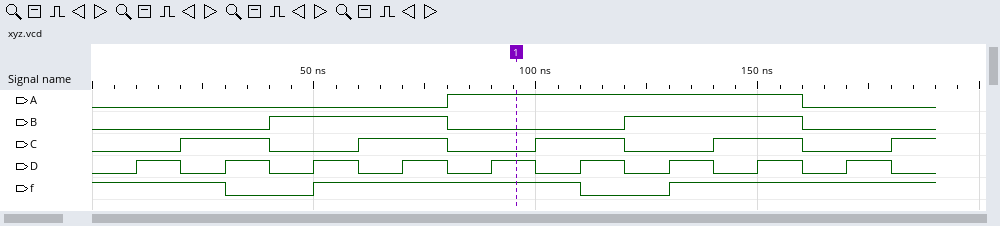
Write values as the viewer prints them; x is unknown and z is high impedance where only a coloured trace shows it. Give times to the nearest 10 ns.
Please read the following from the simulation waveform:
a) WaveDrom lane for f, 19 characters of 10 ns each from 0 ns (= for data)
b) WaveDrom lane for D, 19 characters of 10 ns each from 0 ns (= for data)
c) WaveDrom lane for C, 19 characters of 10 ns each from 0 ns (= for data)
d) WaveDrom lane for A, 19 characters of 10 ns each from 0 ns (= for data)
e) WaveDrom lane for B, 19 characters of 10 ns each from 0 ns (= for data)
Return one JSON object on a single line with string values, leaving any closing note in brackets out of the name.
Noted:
{"WaveDrom lane for f, 19 characters of 10 ns each from 0 ns": "{name: 'f', wave: '1..0.1.....0.1.....'}", "WaveDrom lane for D, 19 characters of 10 ns each from 0 ns": "{name: 'D', wave: '0101010101010101010'}", "WaveDrom lane for C, 19 characters of 10 ns each from 0 ns": "{name: 'C', wave: '0.1.0.1.0.1.0.1.0.1'}", "WaveDrom lane for A, 19 characters of 10 ns each from 0 ns": "{name: 'A', wave: '0.......1.......0..'}", "WaveDrom lane for B, 19 characters of 10 ns each from 0 ns": "{name: 'B', wave: '0...1...0...1...0..'}"}
